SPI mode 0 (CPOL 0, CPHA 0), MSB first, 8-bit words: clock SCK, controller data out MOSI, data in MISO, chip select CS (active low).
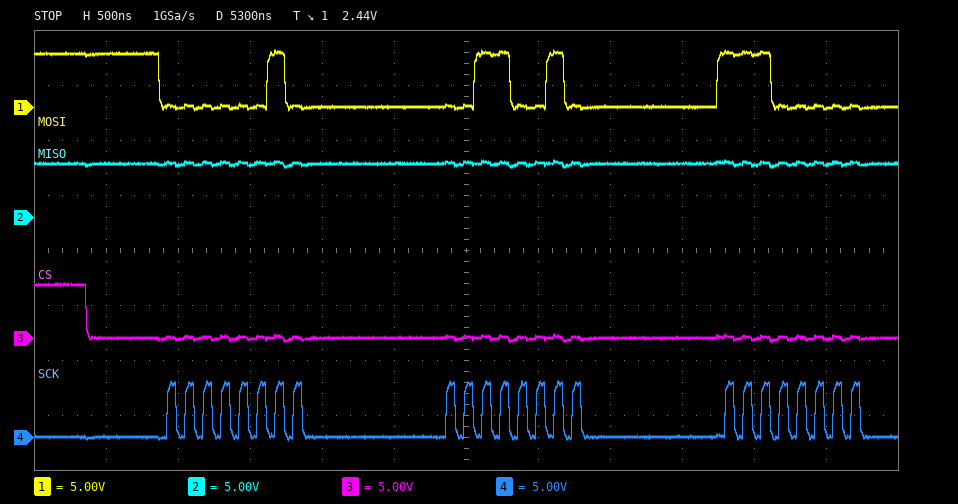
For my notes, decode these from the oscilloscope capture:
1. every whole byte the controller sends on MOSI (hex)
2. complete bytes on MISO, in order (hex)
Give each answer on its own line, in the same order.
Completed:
02 32 E0
FF FF FF
